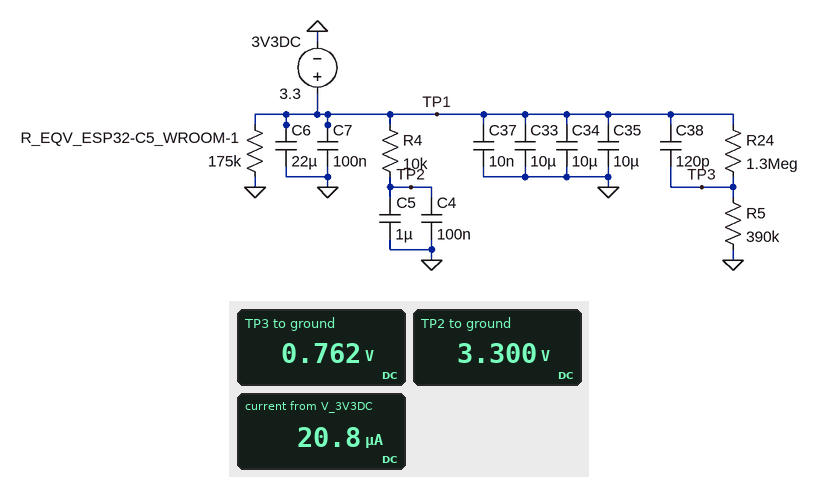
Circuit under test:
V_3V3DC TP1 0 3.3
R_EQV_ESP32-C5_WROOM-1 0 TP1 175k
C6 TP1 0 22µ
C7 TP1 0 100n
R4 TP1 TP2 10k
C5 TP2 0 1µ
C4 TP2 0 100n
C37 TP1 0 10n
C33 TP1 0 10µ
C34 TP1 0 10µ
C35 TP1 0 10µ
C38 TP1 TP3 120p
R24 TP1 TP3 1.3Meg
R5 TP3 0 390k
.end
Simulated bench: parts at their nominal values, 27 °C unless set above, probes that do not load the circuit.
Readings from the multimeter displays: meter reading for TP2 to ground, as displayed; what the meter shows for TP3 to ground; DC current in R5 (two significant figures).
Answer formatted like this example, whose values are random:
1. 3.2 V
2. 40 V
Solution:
1. 3.300 V
2. 0.762 V
3. 2.0 µA
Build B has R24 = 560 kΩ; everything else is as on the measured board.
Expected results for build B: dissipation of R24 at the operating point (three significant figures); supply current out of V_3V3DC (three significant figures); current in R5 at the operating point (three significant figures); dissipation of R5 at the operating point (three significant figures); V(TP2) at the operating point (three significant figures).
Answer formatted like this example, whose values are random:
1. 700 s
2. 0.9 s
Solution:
1. 6.76 µW
2. 22.3 µA
3. 3.47 µA
4. 4.71 µW
5. 3.30 V
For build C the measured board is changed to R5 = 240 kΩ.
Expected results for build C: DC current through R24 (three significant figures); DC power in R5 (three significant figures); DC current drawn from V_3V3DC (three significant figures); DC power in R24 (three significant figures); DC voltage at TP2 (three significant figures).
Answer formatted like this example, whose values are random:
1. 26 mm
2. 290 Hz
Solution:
1. 2.14 µA
2. 1.10 µW
3. 21.0 µA
4. 5.97 µW
5. 3.30 V
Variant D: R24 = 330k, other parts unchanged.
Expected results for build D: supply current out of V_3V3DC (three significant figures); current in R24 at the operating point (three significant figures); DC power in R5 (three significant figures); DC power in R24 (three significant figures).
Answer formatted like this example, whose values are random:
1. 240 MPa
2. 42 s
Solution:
1. 23.4 µA
2. 4.58 µA
3. 8.19 µW
4. 6.93 µW
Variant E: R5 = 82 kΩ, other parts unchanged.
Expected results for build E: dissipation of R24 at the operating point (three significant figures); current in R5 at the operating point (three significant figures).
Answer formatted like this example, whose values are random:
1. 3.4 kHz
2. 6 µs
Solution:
1. 7.41 µW
2. 2.39 µA
